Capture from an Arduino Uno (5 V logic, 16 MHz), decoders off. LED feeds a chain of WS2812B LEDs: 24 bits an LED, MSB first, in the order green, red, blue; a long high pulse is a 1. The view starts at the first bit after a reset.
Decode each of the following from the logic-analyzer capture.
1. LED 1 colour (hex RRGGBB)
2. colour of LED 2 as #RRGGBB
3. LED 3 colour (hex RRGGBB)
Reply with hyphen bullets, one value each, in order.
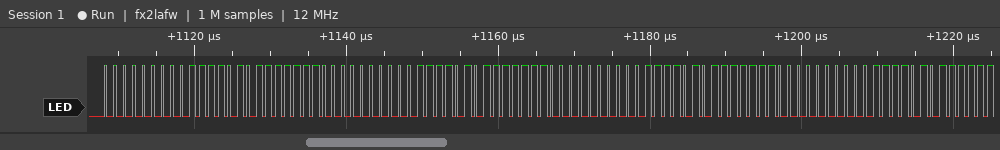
- #7A00FE
- #7A00FE
- #7A00FE
